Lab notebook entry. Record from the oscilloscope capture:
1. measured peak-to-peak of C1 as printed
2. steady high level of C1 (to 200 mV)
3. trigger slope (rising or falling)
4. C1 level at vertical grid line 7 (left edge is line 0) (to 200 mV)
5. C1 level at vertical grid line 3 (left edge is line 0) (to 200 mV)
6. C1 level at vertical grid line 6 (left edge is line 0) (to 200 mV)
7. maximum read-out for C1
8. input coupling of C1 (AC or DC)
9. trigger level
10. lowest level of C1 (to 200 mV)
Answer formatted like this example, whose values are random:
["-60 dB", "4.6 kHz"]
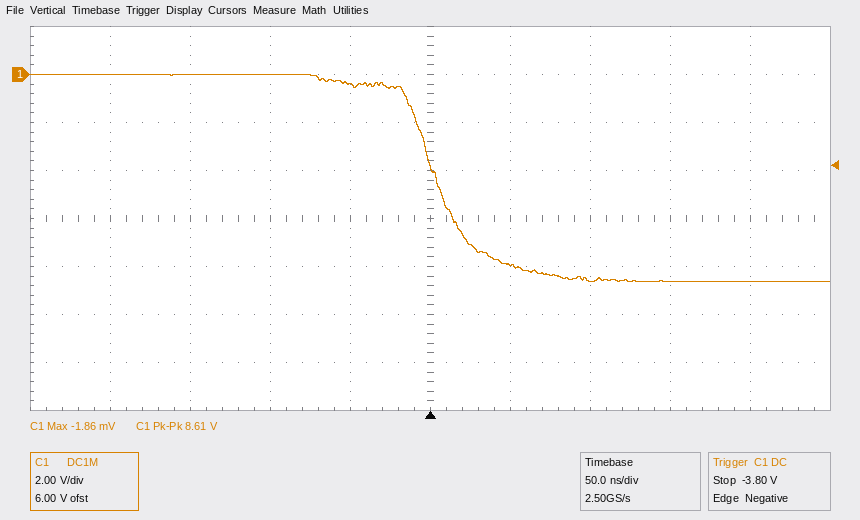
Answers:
["8.61 V", "0.0 V", "falling", "-8.6 V", "0.0 V", "-8.0 V", "-1.86 mV", "DC", "-3.80 V", "-8.6 V"]
